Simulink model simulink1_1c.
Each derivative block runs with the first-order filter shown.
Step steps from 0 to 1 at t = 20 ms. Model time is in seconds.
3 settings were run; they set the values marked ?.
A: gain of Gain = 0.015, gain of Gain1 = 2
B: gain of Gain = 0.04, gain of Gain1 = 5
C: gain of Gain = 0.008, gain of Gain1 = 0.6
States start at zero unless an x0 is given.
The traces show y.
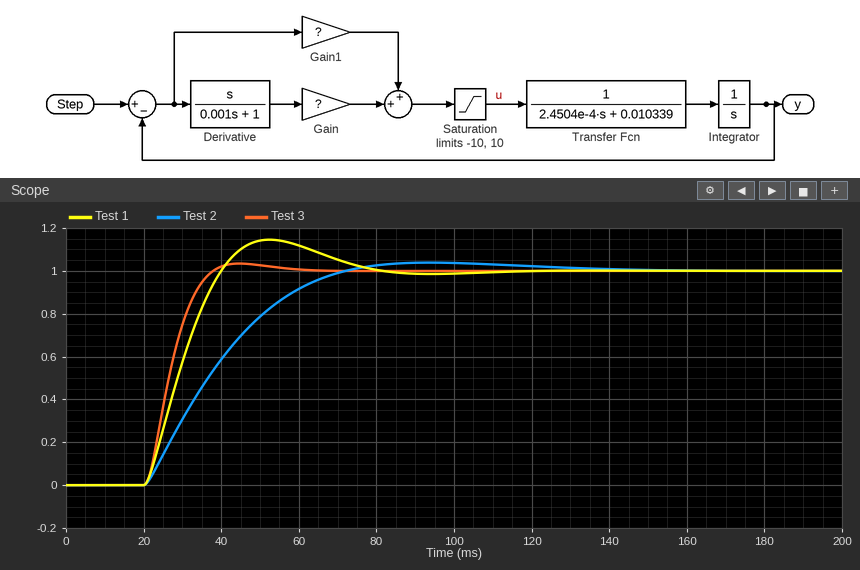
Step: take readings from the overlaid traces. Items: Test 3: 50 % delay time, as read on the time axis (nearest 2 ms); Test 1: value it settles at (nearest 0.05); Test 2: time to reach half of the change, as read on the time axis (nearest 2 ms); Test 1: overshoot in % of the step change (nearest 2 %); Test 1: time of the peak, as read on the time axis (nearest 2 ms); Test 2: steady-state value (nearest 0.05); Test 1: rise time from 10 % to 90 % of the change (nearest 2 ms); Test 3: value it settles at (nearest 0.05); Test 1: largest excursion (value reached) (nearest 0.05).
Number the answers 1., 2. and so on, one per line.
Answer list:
1. 26 ms
2. 1.00
3. 36 ms
4. 14 %
5. 52 ms
6. 1.00
7. 14 ms
8. 1.00
9. 1.15
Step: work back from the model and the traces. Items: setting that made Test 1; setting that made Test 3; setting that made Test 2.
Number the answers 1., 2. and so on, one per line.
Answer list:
1. A
2. B
3. C
